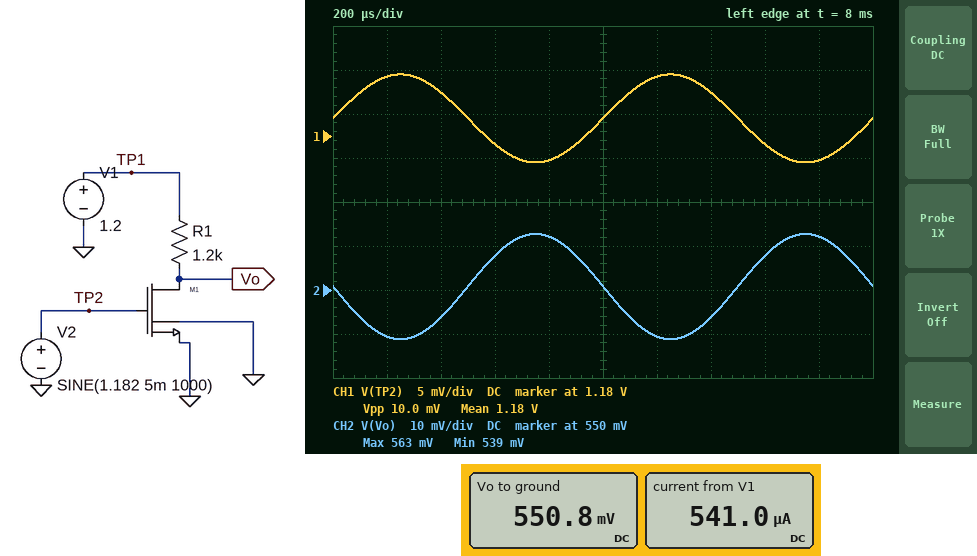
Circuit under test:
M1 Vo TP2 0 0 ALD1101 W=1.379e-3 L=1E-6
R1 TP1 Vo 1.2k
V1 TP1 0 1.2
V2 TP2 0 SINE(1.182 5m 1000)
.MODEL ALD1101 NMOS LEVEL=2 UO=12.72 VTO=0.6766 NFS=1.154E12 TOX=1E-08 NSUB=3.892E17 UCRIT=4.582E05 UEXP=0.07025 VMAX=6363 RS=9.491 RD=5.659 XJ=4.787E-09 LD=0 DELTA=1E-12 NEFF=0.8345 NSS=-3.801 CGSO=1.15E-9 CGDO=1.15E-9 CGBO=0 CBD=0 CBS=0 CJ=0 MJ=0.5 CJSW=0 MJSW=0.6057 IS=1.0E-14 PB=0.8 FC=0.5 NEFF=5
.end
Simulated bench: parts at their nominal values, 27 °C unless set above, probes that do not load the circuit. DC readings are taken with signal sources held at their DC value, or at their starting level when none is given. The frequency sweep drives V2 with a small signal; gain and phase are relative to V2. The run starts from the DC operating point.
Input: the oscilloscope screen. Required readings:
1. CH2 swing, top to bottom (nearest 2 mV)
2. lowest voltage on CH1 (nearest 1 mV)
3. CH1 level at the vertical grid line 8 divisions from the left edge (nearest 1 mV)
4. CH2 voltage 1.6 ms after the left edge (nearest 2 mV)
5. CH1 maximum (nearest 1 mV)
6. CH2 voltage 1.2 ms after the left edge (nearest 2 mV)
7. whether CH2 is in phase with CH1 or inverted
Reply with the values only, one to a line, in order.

24 mV
1.177 V
1.179 V
558 mV
1.187 V
540 mV
inverted
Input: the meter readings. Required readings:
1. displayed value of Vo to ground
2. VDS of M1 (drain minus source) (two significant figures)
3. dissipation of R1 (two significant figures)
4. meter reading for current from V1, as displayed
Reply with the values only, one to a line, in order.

550.8 mV
550 mV
350 µW
541.0 µA
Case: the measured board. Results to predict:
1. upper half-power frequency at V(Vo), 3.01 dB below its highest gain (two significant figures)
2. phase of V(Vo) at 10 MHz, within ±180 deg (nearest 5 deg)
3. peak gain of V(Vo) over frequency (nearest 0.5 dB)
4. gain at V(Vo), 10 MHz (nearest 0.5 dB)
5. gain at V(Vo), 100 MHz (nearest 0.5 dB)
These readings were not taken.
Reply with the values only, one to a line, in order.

110 MHz
170 deg
7.5 dB
7.5 dB
5.0 dB
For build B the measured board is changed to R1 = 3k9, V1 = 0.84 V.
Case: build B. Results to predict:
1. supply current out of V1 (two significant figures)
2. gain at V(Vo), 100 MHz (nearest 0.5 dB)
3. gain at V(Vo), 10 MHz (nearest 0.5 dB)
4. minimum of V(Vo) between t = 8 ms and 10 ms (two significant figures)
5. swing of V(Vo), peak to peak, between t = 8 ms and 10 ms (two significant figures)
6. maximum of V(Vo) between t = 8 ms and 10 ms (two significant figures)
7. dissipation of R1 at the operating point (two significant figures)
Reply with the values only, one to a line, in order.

200 µA
-3.5 dB
-15.5 dB
72 mV
1.5 mV
73 mV
150 µW
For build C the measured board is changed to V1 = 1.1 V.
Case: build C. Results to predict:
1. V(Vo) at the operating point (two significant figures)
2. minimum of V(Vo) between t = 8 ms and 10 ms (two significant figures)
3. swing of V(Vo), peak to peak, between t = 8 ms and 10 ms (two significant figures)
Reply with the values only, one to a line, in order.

450 mV
440 mV
24 mV
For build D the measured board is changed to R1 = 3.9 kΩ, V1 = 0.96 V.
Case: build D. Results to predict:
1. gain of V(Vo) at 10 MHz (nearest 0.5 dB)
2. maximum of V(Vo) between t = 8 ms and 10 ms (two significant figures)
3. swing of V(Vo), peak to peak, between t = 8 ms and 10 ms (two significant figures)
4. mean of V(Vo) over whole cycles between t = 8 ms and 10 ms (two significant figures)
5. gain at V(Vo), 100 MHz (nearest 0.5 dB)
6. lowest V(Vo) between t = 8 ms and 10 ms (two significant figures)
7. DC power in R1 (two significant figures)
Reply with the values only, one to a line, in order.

-14.5 dB
85 mV
1.8 mV
84 mV
-3.0 dB
83 mV
200 µW
